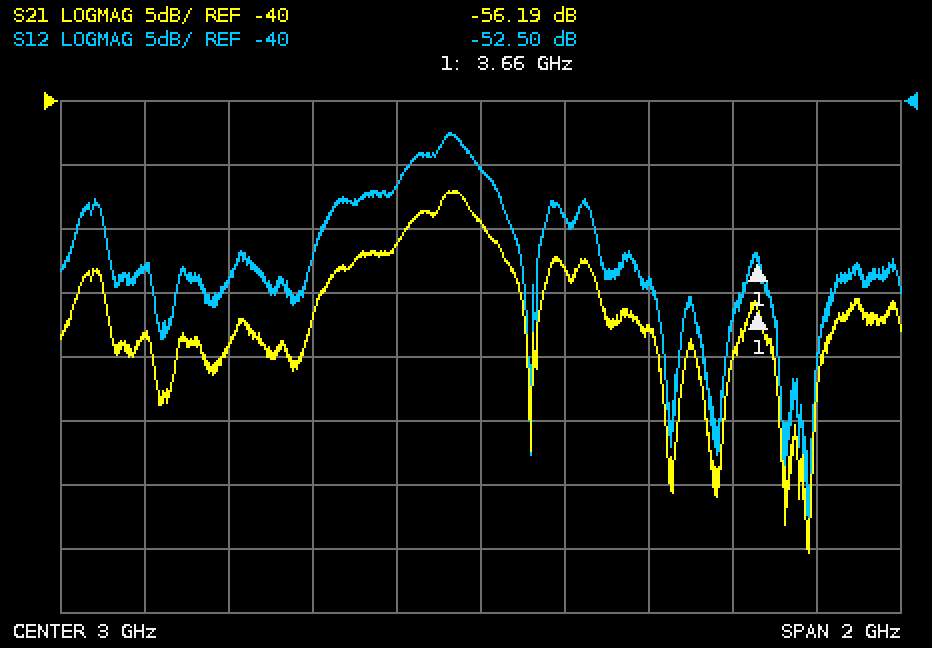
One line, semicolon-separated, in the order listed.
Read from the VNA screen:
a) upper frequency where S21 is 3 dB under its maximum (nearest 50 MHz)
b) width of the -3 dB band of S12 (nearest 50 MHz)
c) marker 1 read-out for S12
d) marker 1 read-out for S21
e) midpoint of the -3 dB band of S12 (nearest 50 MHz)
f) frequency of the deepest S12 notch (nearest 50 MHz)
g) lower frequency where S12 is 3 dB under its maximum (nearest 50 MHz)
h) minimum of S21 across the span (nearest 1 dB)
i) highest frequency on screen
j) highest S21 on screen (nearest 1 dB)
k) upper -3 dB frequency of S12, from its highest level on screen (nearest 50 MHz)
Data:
3.00 GHz; 200 MHz; -52.50 dB; -56.19 dB; 2.90 GHz; 3.80 GHz; 2.80 GHz; -75 dB; 4 GHz; -47 dB; 3.00 GHz
